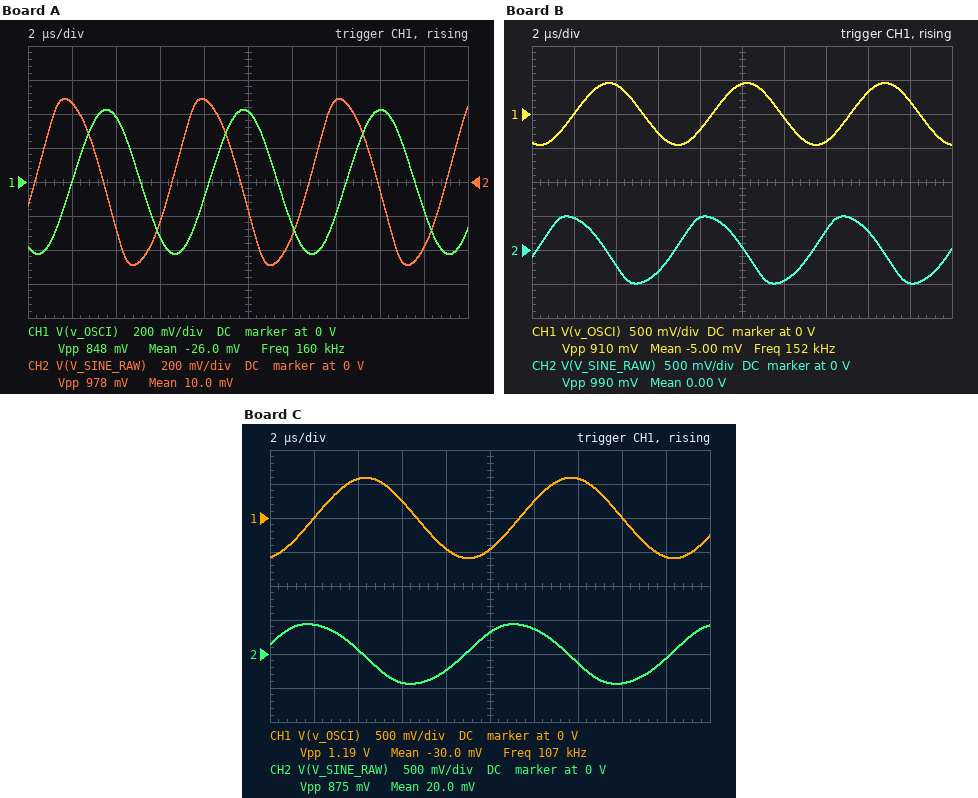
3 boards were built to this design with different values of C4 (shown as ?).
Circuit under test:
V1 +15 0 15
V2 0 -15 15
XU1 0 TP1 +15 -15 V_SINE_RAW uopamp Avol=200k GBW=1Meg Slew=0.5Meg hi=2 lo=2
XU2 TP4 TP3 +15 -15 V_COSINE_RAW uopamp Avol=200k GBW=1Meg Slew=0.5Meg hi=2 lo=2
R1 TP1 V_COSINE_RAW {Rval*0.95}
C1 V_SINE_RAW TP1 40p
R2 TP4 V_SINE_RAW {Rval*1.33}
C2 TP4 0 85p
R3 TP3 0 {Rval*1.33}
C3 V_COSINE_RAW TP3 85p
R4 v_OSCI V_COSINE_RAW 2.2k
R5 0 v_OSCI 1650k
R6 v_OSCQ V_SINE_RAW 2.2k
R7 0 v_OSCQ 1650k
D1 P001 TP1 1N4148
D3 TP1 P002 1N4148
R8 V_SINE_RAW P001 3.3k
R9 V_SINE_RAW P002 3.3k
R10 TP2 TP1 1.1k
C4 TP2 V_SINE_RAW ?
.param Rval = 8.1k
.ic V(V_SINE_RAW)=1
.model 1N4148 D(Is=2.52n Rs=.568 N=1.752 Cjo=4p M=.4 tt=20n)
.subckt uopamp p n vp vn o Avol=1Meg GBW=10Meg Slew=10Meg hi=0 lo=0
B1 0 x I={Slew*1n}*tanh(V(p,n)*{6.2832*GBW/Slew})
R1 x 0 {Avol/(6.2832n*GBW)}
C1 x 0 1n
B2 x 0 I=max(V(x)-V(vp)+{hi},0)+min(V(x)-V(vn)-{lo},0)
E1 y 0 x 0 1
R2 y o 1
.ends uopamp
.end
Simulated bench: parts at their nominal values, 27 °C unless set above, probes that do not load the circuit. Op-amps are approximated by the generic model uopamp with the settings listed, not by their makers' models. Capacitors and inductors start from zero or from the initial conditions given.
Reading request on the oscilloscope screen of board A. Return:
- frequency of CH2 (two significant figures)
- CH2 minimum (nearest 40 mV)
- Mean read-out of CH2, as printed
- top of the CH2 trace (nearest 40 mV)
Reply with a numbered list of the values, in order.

1. 160 kHz
2. -480 mV
3. 10.0 mV
4. 480 mV
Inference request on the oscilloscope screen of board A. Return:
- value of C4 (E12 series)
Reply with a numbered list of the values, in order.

1. 18 pF
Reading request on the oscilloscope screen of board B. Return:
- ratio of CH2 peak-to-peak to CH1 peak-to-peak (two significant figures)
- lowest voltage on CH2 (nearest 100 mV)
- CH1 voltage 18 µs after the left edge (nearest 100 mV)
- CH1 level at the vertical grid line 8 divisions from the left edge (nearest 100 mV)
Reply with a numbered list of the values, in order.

1. 1.1
2. -500 mV
3. 200 mV
4. 300 mV
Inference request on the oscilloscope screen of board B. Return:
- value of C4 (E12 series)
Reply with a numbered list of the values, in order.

1. 33 pF
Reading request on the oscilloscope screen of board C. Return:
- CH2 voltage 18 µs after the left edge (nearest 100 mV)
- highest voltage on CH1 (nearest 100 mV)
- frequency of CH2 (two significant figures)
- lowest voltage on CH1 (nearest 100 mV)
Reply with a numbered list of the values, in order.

1. -100 mV
2. 600 mV
3. 110 kHz
4. -600 mV
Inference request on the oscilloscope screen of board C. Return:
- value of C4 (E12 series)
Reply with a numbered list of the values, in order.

1. 180 pF
